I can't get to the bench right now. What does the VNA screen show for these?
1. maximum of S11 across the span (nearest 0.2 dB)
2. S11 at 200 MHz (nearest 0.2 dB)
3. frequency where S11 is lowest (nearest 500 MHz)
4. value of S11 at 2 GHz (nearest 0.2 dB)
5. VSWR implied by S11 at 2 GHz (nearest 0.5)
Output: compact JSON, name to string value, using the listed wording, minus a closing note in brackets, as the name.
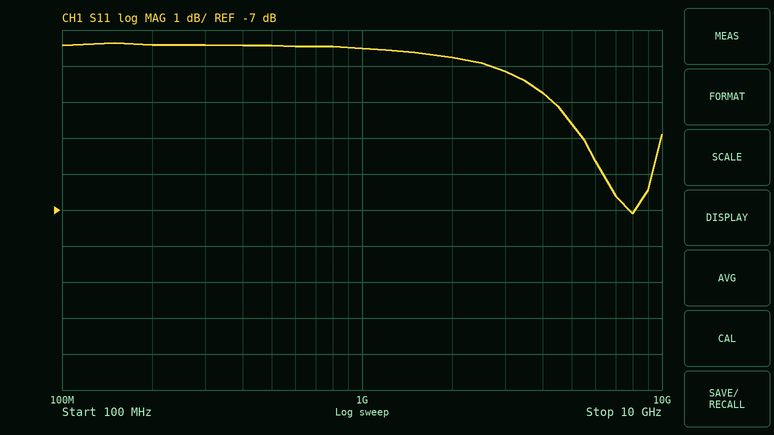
{"maximum of S11 across the span": "-2.4 dB", "S11 at 200 MHz": "-2.4 dB", "frequency where S11 is lowest": "8.0 GHz", "value of S11 at 2 GHz": "-2.8 dB", "VSWR implied by S11 at 2 GHz": "6.5"}
